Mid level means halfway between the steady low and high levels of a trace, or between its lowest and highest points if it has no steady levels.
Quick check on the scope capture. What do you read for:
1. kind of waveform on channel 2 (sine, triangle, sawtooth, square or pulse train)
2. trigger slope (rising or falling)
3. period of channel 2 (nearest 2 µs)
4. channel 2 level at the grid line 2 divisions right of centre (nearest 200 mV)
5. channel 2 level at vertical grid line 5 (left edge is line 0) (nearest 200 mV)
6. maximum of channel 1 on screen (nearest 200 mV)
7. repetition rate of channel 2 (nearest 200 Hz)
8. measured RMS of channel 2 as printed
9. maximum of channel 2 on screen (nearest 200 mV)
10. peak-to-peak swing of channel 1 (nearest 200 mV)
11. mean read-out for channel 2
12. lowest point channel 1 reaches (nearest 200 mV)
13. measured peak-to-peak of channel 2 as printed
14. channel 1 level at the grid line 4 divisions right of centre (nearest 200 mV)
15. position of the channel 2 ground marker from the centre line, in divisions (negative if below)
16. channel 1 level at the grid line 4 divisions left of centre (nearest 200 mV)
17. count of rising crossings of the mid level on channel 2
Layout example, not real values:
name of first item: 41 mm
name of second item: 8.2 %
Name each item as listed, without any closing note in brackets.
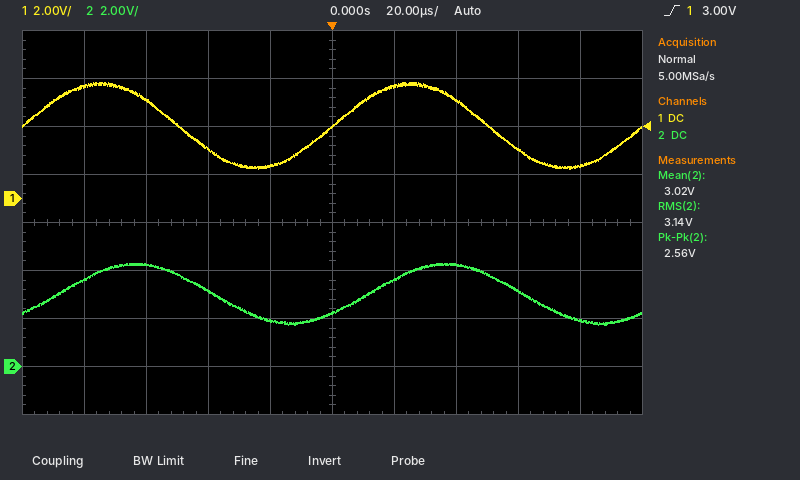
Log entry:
kind of waveform on channel 2: sine
trigger slope: rising
period of channel 2: 100 µs
channel 2 level at the grid line 2 divisions right of centre: 4.2 V
channel 2 level at vertical grid line 5 (left edge is line 0): 2.2 V
maximum of channel 1 on screen: 4.8 V
repetition rate of channel 2: 10.0 kHz
measured RMS of channel 2 as printed: 3.14 V
maximum of channel 2 on screen: 4.2 V
peak-to-peak swing of channel 1: 3.6 V
mean read-out for channel 2: 3.02 V
lowest point channel 1 reaches: 1.2 V
measured peak-to-peak of channel 2 as printed: 2.56 V
channel 1 level at the grid line 4 divisions right of centre: 1.4 V
position of the channel 2 ground marker from the centre line, in divisions: -3.0 div
channel 1 level at the grid line 4 divisions left of centre: 4.6 V
count of rising crossings of the mid level on channel 2: 2
